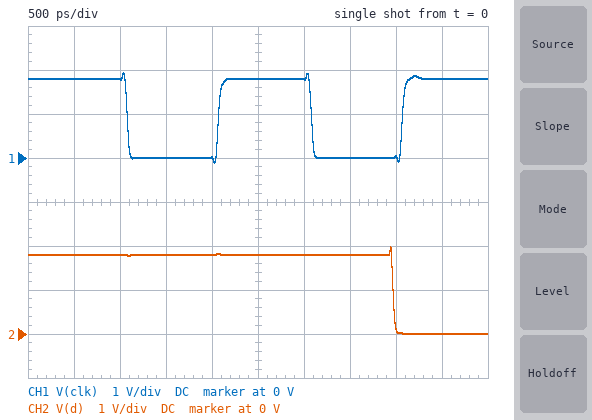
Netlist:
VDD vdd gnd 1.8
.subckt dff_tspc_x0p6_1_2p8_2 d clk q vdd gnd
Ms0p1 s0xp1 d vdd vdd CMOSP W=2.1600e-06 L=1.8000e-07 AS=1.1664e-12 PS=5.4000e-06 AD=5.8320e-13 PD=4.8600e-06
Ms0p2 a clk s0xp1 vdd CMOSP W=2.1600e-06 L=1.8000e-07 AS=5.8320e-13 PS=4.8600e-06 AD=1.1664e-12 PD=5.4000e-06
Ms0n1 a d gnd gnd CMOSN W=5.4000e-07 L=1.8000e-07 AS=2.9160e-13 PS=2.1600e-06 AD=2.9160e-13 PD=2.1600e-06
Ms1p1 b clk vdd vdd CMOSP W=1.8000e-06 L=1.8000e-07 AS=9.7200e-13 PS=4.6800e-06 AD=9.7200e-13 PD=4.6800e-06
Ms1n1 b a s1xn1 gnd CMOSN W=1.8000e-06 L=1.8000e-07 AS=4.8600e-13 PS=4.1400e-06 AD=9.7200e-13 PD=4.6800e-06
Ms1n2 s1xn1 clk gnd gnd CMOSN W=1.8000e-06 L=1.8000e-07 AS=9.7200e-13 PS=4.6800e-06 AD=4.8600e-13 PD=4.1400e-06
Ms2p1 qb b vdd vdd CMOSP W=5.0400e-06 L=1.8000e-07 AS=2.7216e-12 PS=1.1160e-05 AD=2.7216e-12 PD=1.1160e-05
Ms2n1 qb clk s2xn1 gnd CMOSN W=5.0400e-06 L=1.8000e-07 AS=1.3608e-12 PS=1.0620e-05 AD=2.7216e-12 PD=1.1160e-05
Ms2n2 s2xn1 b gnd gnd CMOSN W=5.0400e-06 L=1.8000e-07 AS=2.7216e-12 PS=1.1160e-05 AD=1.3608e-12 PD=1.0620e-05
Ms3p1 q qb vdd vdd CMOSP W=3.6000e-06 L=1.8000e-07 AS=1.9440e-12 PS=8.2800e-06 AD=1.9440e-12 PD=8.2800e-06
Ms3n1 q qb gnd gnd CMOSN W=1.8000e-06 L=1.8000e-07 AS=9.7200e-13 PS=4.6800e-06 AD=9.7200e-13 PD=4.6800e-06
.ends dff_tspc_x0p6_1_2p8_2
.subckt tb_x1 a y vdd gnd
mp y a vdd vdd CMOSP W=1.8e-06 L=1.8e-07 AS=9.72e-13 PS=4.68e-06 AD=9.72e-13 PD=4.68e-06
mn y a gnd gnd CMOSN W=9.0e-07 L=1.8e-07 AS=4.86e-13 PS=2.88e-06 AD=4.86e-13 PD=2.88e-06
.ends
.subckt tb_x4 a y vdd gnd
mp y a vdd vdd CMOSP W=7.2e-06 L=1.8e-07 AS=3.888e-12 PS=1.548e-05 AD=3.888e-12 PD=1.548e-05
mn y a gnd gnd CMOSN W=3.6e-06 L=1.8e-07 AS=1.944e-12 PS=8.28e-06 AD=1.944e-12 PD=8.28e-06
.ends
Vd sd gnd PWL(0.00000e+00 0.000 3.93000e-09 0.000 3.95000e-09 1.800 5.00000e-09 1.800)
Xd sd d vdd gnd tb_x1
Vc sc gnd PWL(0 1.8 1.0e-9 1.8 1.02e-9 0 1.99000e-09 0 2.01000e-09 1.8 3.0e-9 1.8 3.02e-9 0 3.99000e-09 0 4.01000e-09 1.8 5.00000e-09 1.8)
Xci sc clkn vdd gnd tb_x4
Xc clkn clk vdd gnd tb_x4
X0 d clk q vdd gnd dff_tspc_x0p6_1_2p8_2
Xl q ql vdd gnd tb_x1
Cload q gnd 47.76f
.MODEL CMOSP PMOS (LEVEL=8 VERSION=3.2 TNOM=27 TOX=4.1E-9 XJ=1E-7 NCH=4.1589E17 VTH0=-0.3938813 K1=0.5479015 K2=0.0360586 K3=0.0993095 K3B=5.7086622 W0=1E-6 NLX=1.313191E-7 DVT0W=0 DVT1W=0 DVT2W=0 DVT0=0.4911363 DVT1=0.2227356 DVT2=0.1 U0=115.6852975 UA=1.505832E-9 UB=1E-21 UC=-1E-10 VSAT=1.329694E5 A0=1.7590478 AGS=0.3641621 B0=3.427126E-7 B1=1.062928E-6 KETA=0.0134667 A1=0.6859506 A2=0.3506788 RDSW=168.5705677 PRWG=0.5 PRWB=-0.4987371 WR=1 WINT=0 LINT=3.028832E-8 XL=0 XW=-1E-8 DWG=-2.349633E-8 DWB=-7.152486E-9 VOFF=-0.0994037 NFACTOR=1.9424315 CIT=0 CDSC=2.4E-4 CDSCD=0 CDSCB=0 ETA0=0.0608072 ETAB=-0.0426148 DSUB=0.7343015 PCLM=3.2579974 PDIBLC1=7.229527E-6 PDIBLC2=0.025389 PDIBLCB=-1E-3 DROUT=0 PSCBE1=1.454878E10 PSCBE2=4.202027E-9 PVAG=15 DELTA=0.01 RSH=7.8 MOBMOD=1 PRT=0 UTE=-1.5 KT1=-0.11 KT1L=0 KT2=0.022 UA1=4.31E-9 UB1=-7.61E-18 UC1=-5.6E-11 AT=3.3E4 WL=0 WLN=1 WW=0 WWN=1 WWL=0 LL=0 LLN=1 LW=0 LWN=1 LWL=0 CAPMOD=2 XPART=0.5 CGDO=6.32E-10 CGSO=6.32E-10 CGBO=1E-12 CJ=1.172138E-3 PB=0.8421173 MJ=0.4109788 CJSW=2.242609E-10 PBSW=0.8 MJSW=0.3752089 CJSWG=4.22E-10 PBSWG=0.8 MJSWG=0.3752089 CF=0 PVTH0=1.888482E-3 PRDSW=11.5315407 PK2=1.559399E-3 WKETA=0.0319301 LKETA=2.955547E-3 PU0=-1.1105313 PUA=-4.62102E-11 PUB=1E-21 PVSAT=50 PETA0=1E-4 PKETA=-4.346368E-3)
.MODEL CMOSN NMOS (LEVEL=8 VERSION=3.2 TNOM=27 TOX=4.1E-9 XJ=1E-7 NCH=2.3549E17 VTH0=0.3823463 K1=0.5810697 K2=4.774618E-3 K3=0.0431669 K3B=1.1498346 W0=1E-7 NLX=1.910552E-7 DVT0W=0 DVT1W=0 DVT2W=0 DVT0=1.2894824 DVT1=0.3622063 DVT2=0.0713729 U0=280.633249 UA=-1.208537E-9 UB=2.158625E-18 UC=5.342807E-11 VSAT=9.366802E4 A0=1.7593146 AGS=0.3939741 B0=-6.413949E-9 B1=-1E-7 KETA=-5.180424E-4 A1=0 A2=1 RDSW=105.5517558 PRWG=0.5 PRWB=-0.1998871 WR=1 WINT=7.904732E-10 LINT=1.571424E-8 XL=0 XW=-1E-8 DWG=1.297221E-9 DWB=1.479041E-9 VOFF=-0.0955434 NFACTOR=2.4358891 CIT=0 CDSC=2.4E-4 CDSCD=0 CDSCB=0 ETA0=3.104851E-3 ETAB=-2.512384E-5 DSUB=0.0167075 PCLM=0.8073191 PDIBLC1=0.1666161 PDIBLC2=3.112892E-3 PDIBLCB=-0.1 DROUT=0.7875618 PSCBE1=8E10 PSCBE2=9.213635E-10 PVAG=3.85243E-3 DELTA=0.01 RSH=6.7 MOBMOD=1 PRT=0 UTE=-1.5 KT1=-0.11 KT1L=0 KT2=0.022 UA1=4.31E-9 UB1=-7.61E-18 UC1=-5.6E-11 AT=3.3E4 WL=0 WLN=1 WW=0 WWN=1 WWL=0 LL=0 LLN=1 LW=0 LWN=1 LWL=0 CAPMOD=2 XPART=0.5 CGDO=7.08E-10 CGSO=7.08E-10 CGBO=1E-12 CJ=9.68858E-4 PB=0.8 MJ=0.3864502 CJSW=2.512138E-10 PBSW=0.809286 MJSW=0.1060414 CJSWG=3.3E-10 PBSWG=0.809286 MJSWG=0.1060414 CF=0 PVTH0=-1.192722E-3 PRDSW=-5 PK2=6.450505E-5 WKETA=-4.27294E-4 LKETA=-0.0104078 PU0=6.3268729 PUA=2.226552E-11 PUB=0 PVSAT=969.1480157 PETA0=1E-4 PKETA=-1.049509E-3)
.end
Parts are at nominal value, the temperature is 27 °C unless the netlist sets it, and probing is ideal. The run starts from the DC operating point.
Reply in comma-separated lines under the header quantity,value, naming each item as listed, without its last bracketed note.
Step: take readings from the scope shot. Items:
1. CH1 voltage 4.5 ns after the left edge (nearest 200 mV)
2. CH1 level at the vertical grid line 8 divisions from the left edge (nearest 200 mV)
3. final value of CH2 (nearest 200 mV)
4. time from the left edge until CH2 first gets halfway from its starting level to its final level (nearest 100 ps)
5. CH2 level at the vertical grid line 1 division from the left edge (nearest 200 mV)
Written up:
quantity,value
CH1 voltage 4.5 ns after the left edge,1.8 V
CH1 level at the vertical grid line 8 divisions from the left edge,0 V
final value of CH2,0 V
time from the left edge until CH2 first gets halfway from its starting level to its final level,4.0 ns
CH2 level at the vertical grid line 1 division from the left edge,1.8 V
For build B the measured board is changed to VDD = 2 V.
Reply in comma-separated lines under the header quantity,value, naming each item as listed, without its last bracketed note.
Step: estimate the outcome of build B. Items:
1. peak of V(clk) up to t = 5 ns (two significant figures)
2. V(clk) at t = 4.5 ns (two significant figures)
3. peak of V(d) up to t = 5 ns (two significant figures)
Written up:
quantity,value
peak of V(clk) up to t = 5 ns,2.1 V
V(clk) at t = 4.5 ns,2.0 V
peak of V(d) up to t = 5 ns,2.2 V
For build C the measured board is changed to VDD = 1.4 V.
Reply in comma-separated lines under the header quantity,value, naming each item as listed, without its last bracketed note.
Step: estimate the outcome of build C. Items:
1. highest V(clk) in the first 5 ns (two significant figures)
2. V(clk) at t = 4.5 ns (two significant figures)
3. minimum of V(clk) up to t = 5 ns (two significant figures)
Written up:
quantity,value
highest V(clk) in the first 5 ns,1.5 V
V(clk) at t = 4.5 ns,1.4 V
minimum of V(clk) up to t = 5 ns,-140 mV
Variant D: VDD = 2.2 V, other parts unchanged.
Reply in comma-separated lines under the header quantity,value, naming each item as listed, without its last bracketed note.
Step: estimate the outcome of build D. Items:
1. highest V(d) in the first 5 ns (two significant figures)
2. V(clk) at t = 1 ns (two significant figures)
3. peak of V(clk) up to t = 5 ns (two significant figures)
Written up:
quantity,value
highest V(d) in the first 5 ns,2.4 V
V(clk) at t = 1 ns,2.2 V
peak of V(clk) up to t = 5 ns,2.3 V
